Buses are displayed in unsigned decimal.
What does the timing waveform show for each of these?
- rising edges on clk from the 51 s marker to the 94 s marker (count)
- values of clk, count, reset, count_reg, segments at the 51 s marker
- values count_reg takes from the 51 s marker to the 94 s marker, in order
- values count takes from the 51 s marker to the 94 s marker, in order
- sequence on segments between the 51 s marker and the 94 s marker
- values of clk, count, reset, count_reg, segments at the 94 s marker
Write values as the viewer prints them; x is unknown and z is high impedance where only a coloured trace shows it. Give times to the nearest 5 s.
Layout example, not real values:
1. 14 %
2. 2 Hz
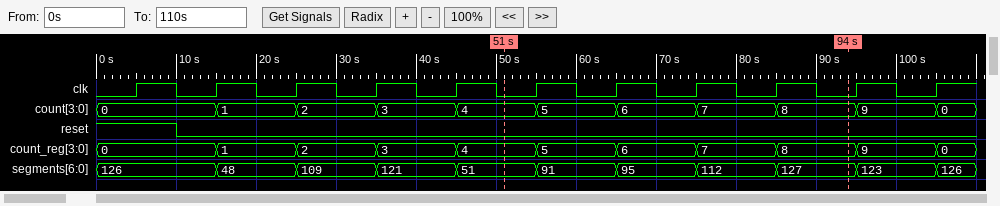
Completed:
1. 4
2. clk=0, count=4, reset=0, count_reg=4, segments=51
3. 4, 5, 6, 7, 8
4. 4, 5, 6, 7, 8
5. 51, 91, 95, 112, 127
6. clk=0, count=8, reset=0, count_reg=8, segments=127
